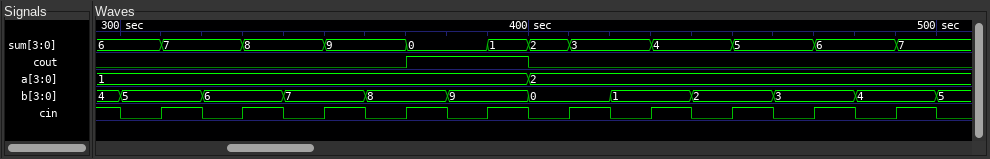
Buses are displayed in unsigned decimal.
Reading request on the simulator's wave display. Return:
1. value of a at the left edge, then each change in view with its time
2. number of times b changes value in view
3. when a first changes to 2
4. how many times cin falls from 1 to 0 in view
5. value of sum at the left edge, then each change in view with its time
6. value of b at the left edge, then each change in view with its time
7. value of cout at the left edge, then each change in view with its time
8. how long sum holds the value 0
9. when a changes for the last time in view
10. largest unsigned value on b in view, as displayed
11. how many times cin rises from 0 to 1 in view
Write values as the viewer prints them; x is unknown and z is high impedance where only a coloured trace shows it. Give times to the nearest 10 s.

1, 2 at 400 s
11
400 s
11
6, 7 at 310 s, 8 at 330 s, 9 at 350 s, 0 at 370 s, 1 at 390 s, 2 at 400 s, 3 at 410 s, 4 at 430 s, 5 at 450 s, 6 at 470 s, 7 at 490 s
4, 5 at 300 s, 6 at 320 s, 7 at 340 s, 8 at 360 s, 9 at 380 s, 0 at 400 s, 1 at 420 s, 2 at 440 s, 3 at 460 s, 4 at 480 s, 5 at 500 s
0, 1 at 370 s, 0 at 400 s
20 s
400 s
9
10
